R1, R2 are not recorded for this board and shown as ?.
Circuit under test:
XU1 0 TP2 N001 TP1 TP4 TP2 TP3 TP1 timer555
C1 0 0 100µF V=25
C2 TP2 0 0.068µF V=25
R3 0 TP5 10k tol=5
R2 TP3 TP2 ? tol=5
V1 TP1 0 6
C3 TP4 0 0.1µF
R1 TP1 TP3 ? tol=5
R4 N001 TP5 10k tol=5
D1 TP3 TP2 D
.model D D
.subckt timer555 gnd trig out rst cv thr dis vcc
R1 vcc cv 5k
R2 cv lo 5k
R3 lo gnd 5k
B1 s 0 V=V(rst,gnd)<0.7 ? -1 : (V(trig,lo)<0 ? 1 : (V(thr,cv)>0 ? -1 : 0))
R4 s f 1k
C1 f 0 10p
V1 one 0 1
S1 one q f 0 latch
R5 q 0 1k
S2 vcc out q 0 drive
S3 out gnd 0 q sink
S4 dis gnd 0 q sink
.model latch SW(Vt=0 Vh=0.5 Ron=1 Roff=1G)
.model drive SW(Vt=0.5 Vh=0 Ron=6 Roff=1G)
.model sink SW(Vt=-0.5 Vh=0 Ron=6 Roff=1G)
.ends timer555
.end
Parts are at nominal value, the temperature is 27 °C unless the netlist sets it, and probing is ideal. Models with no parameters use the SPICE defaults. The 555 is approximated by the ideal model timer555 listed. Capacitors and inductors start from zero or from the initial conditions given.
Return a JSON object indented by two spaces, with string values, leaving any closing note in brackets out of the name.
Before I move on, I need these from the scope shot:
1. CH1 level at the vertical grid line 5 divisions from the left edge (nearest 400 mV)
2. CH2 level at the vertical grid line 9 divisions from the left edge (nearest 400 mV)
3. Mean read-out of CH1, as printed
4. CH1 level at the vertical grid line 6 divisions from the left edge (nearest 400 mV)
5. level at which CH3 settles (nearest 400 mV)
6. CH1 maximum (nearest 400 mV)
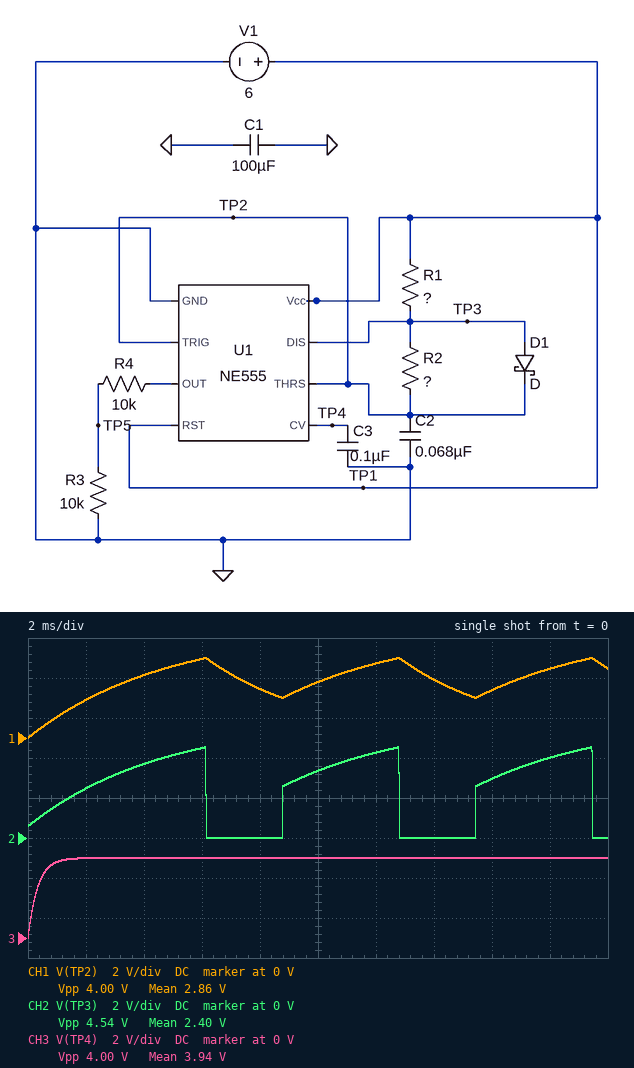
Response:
{
  "CH1 level at the vertical grid line 5 divisions from the left edge": "2.8 V",
  "CH2 level at the vertical grid line 9 divisions from the left edge": "4.0 V",
  "Mean read-out of CH1, as printed": "2.86 V",
  "CH1 level at the vertical grid line 6 divisions from the left edge": "3.6 V",
  "level at which CH3 settles": "4.0 V",
  "CH1 maximum": "4.0 V"
}
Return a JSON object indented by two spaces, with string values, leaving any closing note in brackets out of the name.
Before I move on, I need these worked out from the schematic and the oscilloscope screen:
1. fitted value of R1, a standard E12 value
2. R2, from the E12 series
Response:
{
  "fitted value of R1, a standard E12 value": "68 kΩ",
  "R2, from the E12 series": "56 kΩ"
}
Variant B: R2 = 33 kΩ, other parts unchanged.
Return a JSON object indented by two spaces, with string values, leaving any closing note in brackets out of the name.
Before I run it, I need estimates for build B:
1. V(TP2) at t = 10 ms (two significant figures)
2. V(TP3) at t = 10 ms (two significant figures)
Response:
{
  "V(TP2) at t = 10 ms": "3.4 V",
  "V(TP3) at t = 10 ms": "3.9 V"
}
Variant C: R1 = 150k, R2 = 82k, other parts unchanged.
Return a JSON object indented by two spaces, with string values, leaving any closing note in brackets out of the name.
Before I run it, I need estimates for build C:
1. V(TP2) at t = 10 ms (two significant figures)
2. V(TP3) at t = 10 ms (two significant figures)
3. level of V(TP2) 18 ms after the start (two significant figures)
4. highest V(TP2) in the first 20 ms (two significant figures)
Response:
{
  "V(TP2) at t = 10 ms": "3.4 V",
  "V(TP3) at t = 10 ms": "3.9 V",
  "level of V(TP2) 18 ms after the start": "2.2 V",
  "highest V(TP2) in the first 20 ms": "4.0 V"
}
